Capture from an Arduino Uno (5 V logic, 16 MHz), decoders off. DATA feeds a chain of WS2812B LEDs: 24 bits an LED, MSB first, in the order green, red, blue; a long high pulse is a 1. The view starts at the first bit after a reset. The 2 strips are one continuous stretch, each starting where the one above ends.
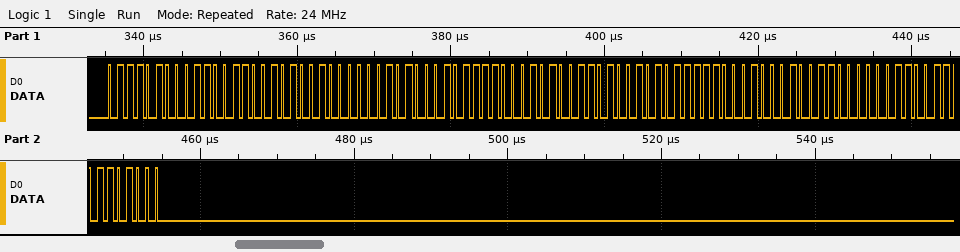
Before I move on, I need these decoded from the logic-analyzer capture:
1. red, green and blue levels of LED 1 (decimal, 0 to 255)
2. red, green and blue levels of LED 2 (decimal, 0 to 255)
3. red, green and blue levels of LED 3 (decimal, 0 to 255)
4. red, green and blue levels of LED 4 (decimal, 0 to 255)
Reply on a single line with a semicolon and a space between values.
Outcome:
102, 116, 82; 23, 5, 138; 95, 105, 17; 51, 48, 104
